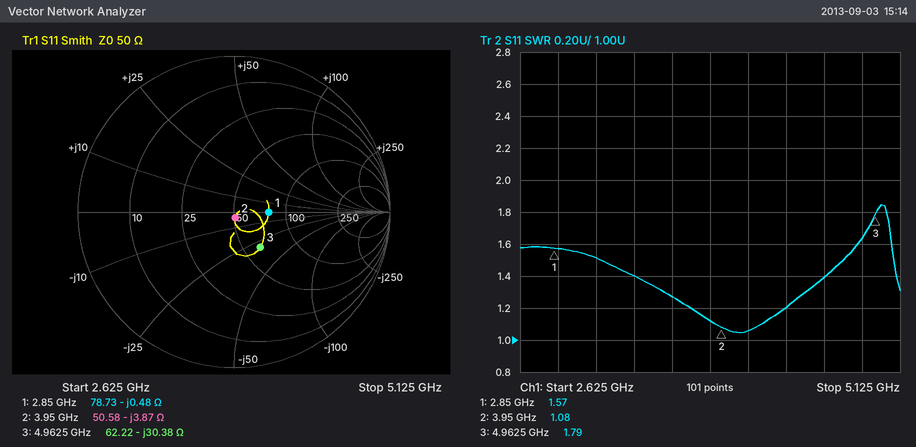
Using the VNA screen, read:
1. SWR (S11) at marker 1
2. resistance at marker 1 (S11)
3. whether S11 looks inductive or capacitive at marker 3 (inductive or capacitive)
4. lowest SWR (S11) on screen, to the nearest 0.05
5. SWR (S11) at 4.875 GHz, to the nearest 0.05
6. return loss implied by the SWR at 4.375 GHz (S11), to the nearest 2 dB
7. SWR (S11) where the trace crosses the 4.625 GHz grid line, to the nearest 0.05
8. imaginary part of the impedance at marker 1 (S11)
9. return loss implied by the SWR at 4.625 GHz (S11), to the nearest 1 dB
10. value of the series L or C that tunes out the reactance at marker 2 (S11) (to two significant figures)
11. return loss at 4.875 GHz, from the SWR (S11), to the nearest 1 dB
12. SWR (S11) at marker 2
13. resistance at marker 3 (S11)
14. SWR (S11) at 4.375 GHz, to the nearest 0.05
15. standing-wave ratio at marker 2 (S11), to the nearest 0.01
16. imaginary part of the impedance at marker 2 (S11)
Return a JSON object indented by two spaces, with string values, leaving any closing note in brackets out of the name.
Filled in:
{
  "SWR (S11) at marker 1": "1.57",
  "resistance at marker 1": "78.73 Ω",
  "whether S11 looks inductive or capacitive at marker 3": "capacitive",
  "lowest SWR (S11) on screen, to the nearest 0.05": "1.05",
  "SWR (S11) at 4.875 GHz, to the nearest 0.05": "1.65",
  "return loss implied by the SWR at 4.375 GHz (S11), to the nearest 2 dB": "20 dB",
  "SWR (S11) where the trace crosses the 4.625 GHz grid line, to the nearest 0.05": "1.40",
  "imaginary part of the impedance at marker 1": "-0.48 Ω",
  "return loss implied by the SWR at 4.625 GHz (S11), to the nearest 1 dB": "16 dB",
  "value of the series L or C that tunes out the reactance at marker 2 (S11)": "160 pH",
  "return loss at 4.875 GHz, from the SWR (S11), to the nearest 1 dB": "12 dB",
  "SWR (S11) at marker 2": "1.08",
  "resistance at marker 3": "62.22 Ω",
  "SWR (S11) at 4.375 GHz, to the nearest 0.05": "1.20",
  "standing-wave ratio at marker 2 (S11), to the nearest 0.01": "1.08",
  "imaginary part of the impedance at marker 2": "-3.87 Ω"
}
